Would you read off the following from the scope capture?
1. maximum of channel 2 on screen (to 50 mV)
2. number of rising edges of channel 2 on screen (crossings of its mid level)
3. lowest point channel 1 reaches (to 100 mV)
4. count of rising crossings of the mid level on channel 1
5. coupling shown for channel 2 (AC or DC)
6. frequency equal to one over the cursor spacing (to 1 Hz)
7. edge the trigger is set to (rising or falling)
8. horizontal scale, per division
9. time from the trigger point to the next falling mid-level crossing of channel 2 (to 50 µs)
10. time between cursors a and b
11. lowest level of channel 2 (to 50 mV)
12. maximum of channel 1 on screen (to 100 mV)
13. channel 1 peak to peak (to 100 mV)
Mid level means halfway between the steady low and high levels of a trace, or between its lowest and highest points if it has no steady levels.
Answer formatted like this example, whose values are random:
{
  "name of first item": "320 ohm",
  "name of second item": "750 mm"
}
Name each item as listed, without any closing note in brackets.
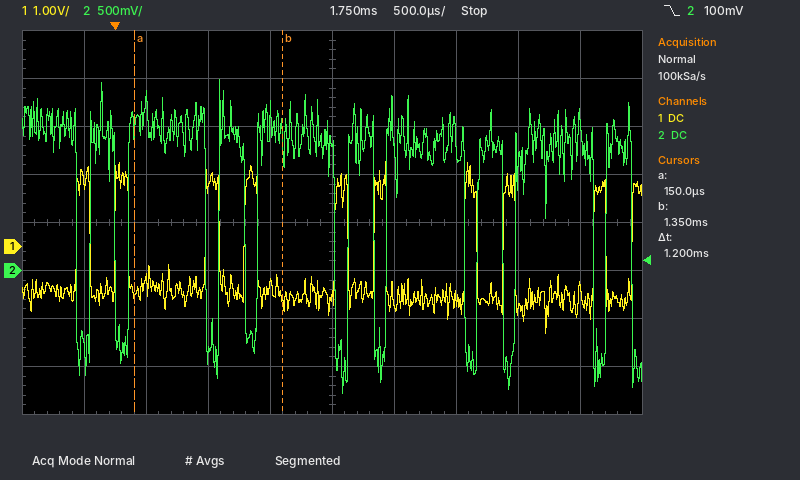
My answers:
{
  "maximum of channel 2 on screen": "2.00 V",
  "number of rising edges of channel 2 on screen": "9",
  "lowest point channel 1 reaches": "-1.8 V",
  "count of rising crossings of the mid level on channel 1": "10",
  "coupling shown for channel 2": "DC",
  "frequency equal to one over the cursor spacing": "833 Hz",
  "edge the trigger is set to": "falling",
  "horizontal scale, per division": "500 µs",
  "time from the trigger point to the next falling mid-level crossing of channel 2": "750 µs",
  "time between cursors a and b": "1.2 ms",
  "lowest level of channel 2": "-1.30 V",
  "maximum of channel 1 on screen": "1.8 V",
  "channel 1 peak to peak": "3.6 V"
}
